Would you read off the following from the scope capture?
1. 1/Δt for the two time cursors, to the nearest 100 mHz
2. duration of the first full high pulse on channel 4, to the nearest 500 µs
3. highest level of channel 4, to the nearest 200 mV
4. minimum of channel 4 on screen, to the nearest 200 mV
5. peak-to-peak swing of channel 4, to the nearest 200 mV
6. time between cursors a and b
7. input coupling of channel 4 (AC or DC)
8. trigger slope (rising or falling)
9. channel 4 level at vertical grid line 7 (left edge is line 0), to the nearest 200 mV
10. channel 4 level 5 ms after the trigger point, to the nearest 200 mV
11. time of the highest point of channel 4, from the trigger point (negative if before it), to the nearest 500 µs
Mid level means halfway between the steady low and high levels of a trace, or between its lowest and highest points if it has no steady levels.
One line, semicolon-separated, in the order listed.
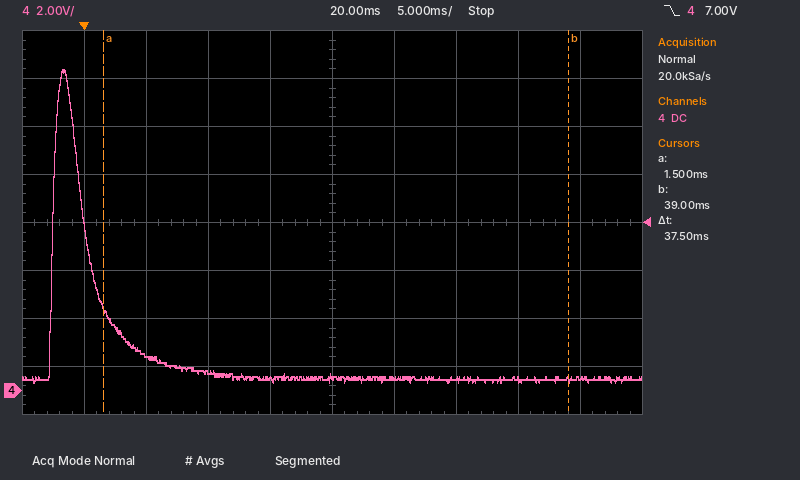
26.7 Hz; 2.5 ms; 13.4 V; 400 mV; 13.0 V; 37.5 ms; DC; falling; 400 mV; 1.4 V; -1.5 ms
